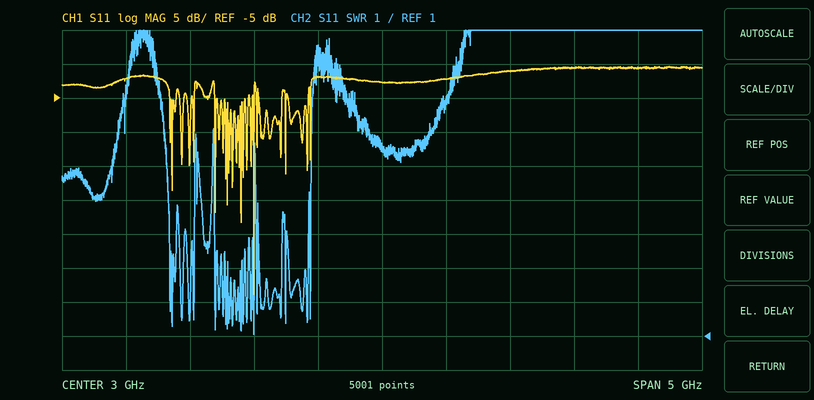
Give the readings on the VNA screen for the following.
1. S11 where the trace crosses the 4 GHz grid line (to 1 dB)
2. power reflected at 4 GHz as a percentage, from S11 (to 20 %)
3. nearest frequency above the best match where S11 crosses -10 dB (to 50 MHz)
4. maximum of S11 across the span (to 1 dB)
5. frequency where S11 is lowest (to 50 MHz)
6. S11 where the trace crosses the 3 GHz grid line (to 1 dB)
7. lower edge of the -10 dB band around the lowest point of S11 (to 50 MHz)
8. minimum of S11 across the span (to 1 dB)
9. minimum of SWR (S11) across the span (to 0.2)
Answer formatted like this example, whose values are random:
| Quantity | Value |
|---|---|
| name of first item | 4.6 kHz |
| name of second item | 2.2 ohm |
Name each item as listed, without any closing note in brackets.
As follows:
| Quantity | Value |
|---|---|
| S11 where the trace crosses the 4 GHz grid line | -1 dB |
| power reflected at 4 GHz as a percentage, from S11 | 80 % |
| nearest frequency above the best match where S11 crosses -10 dB | 2.00 GHz |
| maximum of S11 across the span | 0 dB |
| frequency where S11 is lowest | 2.00 GHz |
| S11 where the trace crosses the 3 GHz grid line | -3 dB |
| lower edge of the -10 dB band around the lowest point of S11 | 2.00 GHz |
| minimum of S11 across the span | -34 dB |
| minimum of SWR (S11) across the span | 1.0 |
